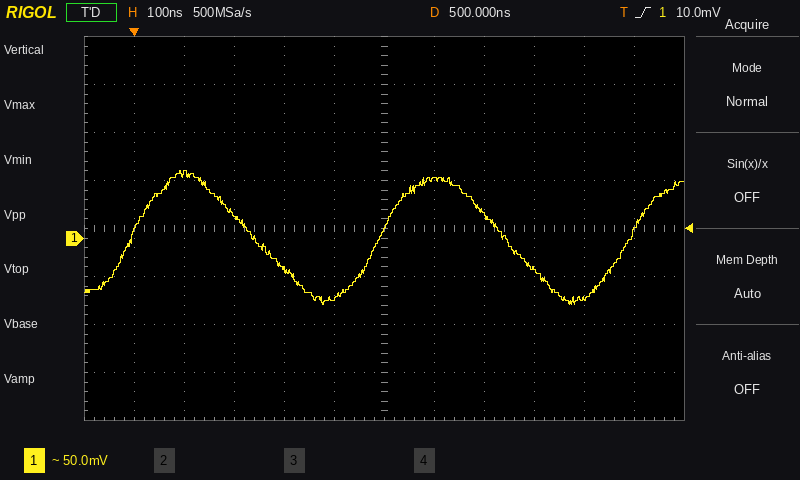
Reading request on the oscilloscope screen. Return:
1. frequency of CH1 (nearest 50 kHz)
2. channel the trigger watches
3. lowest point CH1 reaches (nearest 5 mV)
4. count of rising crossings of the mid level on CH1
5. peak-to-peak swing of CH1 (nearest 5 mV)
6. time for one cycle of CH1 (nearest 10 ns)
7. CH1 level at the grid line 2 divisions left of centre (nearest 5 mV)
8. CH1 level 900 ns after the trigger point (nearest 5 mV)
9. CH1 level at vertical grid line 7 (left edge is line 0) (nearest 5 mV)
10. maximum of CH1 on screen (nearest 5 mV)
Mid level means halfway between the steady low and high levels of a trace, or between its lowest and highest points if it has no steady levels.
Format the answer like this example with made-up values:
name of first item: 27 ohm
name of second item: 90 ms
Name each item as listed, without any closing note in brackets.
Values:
frequency of CH1: 2.00 MHz
channel the trigger watches: CH1
lowest point CH1 reaches: -70 mV
count of rising crossings of the mid level on CH1: 3
peak-to-peak swing of CH1: 140 mV
time for one cycle of CH1: 500 ns
CH1 level at the grid line 2 divisions left of centre: -35 mV
CH1 level 900 ns after the trigger point: -65 mV
CH1 level at vertical grid line 7 (left edge is line 0): 60 mV
maximum of CH1 on screen: 70 mV
